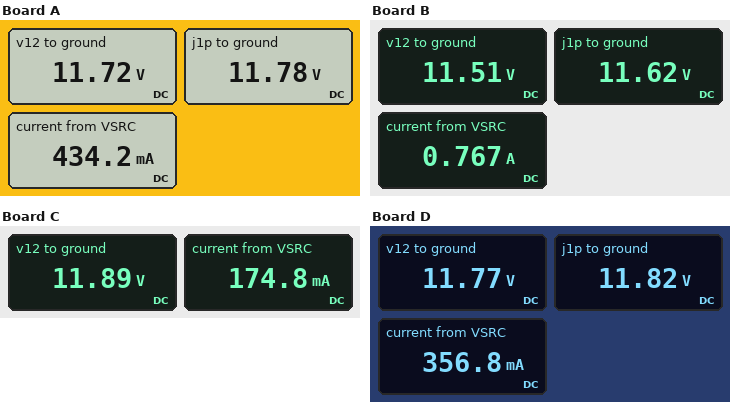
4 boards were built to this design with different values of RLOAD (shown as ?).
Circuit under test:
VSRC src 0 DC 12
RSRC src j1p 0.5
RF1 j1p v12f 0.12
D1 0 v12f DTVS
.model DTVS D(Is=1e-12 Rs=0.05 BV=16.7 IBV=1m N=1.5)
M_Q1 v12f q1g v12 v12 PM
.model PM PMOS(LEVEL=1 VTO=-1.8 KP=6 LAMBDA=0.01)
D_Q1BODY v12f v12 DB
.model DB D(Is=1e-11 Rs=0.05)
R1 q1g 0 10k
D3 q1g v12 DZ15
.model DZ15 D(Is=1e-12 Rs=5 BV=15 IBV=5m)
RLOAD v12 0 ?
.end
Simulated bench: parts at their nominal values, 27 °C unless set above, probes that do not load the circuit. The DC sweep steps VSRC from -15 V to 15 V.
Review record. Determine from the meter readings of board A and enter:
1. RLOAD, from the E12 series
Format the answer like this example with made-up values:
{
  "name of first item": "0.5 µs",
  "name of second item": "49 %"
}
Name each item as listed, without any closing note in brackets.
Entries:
{
  "RLOAD, from the E12 series": "27 Ω"
}
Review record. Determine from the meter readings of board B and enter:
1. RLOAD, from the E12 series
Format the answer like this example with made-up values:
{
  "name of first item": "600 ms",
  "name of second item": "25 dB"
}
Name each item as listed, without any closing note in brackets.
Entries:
{
  "RLOAD, from the E12 series": "15 Ω"
}
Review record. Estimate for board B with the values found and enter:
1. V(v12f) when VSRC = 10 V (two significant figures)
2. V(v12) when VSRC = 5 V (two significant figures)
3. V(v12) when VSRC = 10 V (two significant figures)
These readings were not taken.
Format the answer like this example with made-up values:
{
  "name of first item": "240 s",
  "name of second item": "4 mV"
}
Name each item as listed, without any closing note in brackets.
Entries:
{
  "V(v12f) when VSRC = 10 V": "9.6 V",
  "V(v12) when VSRC = 5 V": "4.8 V",
  "V(v12) when VSRC = 10 V": "9.6 V"
}
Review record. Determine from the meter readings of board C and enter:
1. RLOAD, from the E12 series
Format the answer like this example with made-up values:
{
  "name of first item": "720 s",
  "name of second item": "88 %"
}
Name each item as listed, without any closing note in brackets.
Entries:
{
  "RLOAD, from the E12 series": "68 Ω"
}
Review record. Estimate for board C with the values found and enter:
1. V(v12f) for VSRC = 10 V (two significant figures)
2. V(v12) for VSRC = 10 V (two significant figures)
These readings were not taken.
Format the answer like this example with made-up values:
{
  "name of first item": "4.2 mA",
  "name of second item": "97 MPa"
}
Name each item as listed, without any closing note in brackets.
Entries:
{
  "V(v12f) for VSRC = 10 V": "9.9 V",
  "V(v12) for VSRC = 10 V": "9.9 V"
}
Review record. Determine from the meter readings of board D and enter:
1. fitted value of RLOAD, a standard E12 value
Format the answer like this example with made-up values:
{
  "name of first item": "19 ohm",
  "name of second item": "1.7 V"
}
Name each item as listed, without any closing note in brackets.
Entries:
{
  "fitted value of RLOAD, a standard E12 value": "33 Ω"
}
